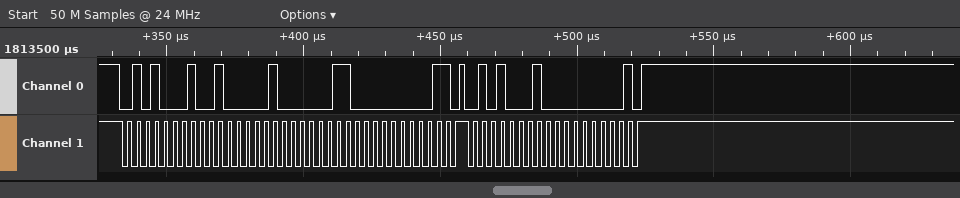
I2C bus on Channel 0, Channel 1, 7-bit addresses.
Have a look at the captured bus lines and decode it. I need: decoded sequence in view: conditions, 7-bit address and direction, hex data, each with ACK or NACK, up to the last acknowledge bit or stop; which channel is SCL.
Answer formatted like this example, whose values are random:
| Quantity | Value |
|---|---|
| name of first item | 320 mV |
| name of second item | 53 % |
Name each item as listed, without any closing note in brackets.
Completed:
| Quantity | Value |
|---|---|
| decoded sequence in view: conditions, 7-bit address and direction, hex data, each with ACK or NACK, up to the last acknowledge bit or stop | start, address 28 read ACK, 41 ACK, 06 ACK, 01 NACK, stop, start, address 28 read ACK, 00 NACK, stop |
| which channel is SCL | Channel 1 |
